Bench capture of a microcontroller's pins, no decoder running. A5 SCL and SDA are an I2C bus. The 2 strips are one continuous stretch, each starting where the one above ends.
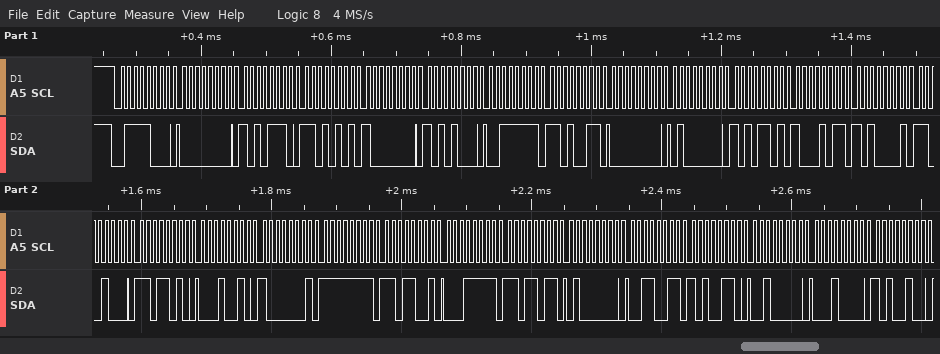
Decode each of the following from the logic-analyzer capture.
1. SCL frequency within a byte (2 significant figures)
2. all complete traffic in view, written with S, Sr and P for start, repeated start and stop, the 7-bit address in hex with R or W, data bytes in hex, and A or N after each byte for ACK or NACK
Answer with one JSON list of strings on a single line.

["100 kHz", "S 3CW A 00 A AE A D5 A 80 A A8 A 3F A D3 A 00 A 40 A AD A 8B A A1 A C8 A DA A 12 A 81 A FF A D9 A 1F A DB A 40 A 33 A A6 A 20 A 10 A A4 A"]
